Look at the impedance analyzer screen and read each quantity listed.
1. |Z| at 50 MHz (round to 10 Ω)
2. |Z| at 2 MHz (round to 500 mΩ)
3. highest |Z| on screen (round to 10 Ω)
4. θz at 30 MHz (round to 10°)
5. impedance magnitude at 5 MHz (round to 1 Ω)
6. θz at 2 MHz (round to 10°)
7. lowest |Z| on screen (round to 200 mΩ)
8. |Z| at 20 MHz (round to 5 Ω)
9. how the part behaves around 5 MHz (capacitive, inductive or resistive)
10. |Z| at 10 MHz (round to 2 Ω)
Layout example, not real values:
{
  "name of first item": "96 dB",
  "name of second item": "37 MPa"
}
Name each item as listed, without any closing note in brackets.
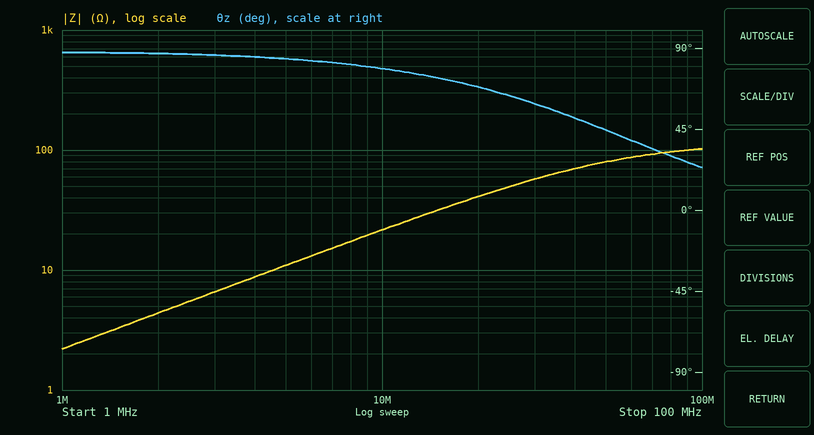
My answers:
{
  "|Z| at 50 MHz": "80 Ω",
  "|Z| at 2 MHz": "4.5 Ω",
  "highest |Z| on screen": "100 Ω",
  "θz at 30 MHz": "60°",
  "impedance magnitude at 5 MHz": "11 Ω",
  "θz at 2 MHz": "90°",
  "lowest |Z| on screen": "2.2 Ω",
  "|Z| at 20 MHz": "40 Ω",
  "how the part behaves around 5 MHz": "inductive",
  "|Z| at 10 MHz": "22 Ω"
}
